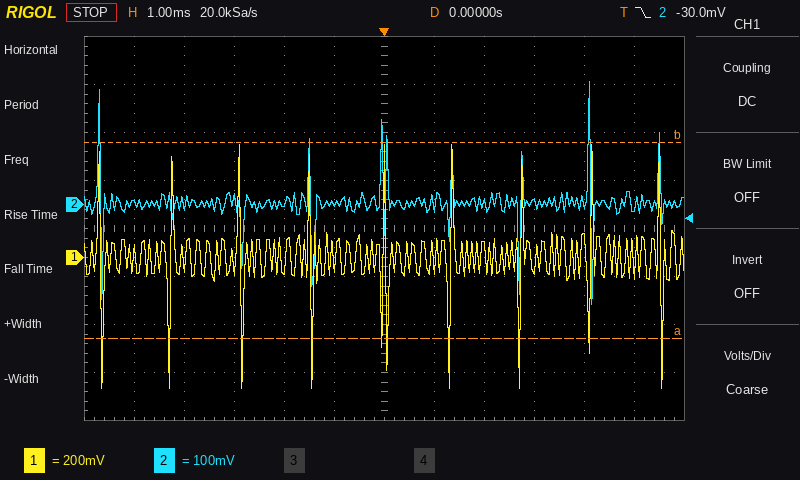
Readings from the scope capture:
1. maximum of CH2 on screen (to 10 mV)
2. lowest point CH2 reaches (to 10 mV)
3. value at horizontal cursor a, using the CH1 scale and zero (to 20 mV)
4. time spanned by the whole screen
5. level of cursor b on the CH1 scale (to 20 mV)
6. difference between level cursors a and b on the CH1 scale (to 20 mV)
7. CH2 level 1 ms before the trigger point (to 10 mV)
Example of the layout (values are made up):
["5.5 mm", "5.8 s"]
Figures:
["260 mV", "-210 mV", "-340 mV", "12 ms", "480 mV", "820 mV", "0 mV"]
